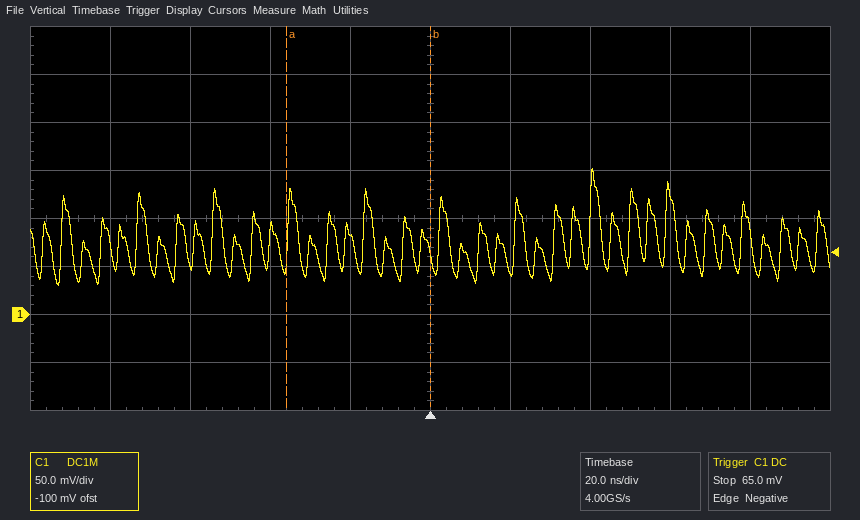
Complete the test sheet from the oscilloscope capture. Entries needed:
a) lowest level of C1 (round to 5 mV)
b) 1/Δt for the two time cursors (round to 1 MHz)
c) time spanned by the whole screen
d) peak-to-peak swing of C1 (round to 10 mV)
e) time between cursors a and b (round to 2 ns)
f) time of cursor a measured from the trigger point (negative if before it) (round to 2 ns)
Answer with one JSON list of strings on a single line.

["30 mV", "28 MHz", "200 ns", "120 mV", "36 ns", "-36 ns"]
